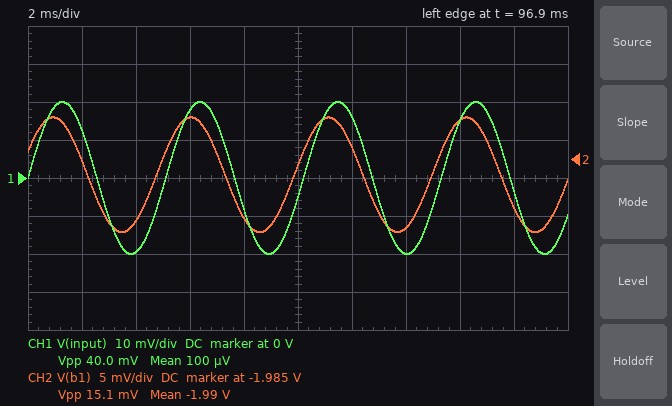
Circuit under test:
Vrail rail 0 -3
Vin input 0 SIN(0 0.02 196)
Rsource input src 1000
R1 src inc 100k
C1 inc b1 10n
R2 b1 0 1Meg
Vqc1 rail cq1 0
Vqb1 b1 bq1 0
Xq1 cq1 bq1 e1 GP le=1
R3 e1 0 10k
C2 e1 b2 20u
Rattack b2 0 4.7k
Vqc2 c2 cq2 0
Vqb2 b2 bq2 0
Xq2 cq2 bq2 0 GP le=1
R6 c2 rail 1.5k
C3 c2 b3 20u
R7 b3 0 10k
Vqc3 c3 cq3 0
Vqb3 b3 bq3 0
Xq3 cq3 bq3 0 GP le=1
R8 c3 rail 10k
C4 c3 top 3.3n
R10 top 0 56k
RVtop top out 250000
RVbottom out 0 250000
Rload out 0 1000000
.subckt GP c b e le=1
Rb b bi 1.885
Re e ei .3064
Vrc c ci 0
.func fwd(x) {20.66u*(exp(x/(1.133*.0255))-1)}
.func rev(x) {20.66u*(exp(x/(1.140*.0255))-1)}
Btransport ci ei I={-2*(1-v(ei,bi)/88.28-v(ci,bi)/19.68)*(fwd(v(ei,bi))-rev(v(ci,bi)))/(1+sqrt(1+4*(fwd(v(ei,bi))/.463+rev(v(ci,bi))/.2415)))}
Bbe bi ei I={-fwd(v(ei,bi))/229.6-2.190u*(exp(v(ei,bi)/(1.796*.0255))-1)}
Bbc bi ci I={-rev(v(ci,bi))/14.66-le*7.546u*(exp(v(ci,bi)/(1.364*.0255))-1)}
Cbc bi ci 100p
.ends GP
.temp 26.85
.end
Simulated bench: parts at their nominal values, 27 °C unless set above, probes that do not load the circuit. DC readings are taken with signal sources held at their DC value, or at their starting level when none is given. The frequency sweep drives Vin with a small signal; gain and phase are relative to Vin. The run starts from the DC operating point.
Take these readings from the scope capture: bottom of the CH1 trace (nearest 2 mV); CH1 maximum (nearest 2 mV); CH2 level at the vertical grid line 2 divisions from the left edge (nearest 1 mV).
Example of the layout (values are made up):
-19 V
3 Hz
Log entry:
-20 mV
20 mV
-1.993 V
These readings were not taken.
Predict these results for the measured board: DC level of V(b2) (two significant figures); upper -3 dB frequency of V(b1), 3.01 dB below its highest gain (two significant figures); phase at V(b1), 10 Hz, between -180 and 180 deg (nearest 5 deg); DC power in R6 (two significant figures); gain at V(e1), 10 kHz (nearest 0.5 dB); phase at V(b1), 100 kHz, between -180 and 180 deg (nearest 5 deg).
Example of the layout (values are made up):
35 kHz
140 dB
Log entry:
-31 mV
34 kHz
75 deg
9.3 µW
-8.5 dB
-70 deg
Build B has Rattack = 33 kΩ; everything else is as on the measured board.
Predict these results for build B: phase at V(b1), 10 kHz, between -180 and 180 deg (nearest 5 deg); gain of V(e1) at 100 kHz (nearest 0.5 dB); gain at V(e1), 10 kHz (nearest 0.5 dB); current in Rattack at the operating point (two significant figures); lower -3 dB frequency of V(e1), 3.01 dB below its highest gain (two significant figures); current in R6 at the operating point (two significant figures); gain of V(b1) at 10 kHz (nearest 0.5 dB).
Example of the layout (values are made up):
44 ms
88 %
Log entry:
-20 deg
-18.0 dB
-8.0 dB
1.9 µA
85 Hz
210 µA
-7.5 dB
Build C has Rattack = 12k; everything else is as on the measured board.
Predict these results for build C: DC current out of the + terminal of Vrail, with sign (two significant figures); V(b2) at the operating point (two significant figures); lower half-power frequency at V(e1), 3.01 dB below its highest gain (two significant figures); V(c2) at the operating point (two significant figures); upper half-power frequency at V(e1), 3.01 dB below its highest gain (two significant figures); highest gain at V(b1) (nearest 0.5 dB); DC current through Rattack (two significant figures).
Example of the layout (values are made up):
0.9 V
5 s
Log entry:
-460 µA
-50 mV
85 Hz
-2.8 V
29 kHz
-7.0 dB
4.2 µA
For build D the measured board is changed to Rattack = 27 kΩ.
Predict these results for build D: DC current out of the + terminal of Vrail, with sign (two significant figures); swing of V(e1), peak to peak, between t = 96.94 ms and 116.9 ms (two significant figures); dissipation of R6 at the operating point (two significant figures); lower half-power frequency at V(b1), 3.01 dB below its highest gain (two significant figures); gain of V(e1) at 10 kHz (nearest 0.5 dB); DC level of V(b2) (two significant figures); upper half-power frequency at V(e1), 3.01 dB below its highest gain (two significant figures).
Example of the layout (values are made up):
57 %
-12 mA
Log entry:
-520 µA
16 mV
60 µW
85 Hz
-8.0 dB
-61 mV
27 kHz
